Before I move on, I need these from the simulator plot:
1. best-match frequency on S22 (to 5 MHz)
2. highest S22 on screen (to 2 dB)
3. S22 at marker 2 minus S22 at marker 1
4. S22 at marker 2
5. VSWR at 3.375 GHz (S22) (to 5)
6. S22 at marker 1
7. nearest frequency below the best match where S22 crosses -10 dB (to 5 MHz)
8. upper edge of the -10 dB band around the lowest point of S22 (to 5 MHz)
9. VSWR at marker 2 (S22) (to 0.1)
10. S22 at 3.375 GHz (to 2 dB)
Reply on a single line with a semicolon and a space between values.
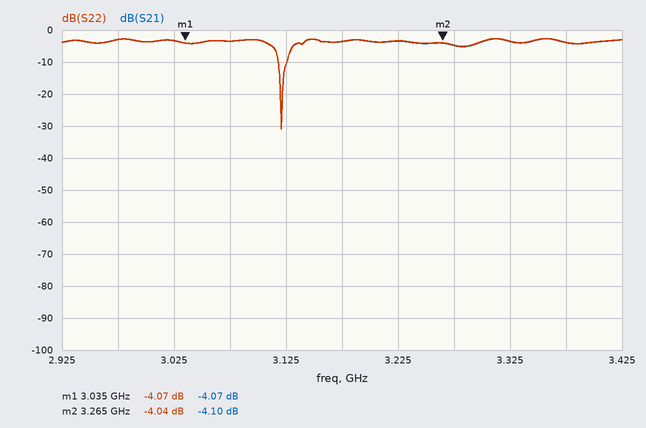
3.120 GHz; -2 dB; 0.03 dB; -4.04 dB; 5; -4.07 dB; 3.120 GHz; 3.125 GHz; 4.4; -4 dB
